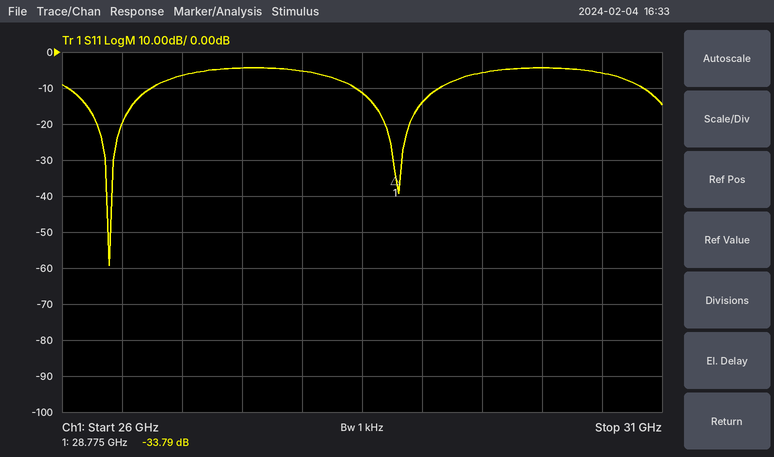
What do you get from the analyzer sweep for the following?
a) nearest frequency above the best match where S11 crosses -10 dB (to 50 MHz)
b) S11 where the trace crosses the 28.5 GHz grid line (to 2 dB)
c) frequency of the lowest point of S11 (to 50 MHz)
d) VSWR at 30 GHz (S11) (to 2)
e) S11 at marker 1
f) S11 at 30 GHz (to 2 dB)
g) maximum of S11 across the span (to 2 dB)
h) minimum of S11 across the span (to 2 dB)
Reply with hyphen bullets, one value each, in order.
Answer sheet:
- 26.75 GHz
- -12 dB
- 26.40 GHz
- 4
- -33.79 dB
- -4 dB
- -4 dB
- -60 dB
